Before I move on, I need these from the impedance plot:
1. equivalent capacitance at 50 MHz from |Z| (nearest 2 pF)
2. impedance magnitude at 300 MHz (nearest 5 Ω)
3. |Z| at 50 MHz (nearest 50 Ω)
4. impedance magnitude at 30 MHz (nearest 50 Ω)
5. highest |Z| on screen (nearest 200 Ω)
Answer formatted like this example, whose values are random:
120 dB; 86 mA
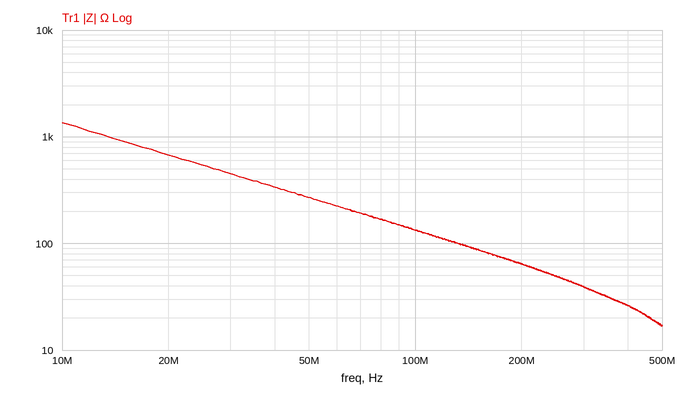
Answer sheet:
12 pF; 40 Ω; 250 Ω; 450 Ω; 1.4 kΩ
